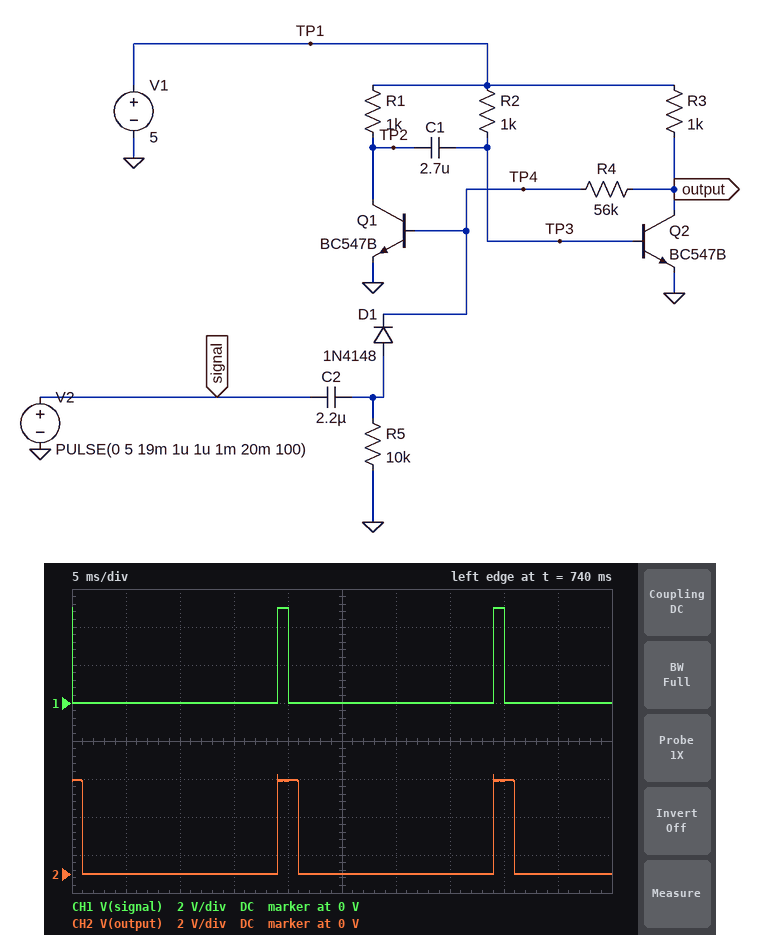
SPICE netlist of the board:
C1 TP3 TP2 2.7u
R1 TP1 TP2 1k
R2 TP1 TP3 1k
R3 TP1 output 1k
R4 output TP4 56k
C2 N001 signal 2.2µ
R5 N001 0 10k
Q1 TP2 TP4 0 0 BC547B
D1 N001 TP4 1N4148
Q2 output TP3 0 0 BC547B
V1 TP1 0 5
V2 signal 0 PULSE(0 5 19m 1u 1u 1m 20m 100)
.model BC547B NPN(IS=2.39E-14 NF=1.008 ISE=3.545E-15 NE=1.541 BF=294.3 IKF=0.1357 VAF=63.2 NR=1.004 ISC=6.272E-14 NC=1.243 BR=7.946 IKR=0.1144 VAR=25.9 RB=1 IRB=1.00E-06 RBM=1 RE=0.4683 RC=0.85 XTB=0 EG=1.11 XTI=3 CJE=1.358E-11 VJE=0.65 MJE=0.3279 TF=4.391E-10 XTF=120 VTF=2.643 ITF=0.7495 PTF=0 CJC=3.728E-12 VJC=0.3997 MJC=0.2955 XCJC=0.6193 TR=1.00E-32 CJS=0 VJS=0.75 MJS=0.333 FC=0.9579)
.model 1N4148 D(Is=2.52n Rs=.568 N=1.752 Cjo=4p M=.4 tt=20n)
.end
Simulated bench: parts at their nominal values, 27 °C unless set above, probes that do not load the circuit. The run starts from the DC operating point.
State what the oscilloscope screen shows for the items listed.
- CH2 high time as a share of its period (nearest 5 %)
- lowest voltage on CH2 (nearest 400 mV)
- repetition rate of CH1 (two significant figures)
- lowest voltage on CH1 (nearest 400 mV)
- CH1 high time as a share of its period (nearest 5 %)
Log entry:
10 %
0 V
50 Hz
0 V
5 %
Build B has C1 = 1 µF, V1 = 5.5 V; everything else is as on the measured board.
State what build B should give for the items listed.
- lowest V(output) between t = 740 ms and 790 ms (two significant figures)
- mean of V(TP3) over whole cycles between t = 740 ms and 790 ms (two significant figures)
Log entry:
22 mV
660 mV
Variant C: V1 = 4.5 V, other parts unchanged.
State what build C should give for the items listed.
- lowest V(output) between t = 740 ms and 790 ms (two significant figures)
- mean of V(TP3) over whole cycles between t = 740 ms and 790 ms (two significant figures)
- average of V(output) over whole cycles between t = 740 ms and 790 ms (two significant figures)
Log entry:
20 mV
540 mV
460 mV
